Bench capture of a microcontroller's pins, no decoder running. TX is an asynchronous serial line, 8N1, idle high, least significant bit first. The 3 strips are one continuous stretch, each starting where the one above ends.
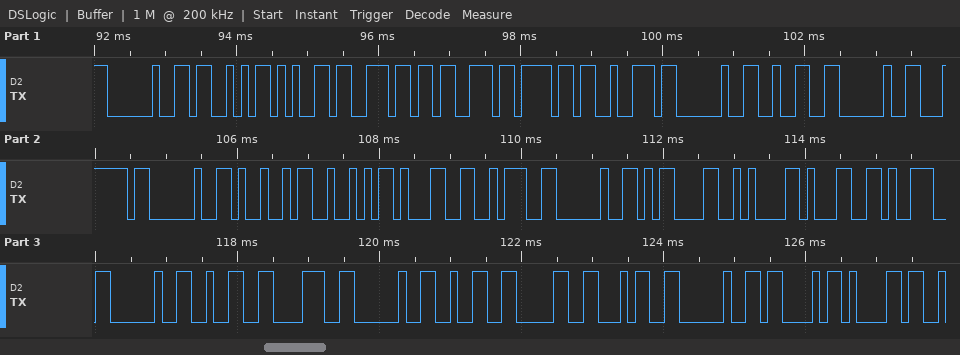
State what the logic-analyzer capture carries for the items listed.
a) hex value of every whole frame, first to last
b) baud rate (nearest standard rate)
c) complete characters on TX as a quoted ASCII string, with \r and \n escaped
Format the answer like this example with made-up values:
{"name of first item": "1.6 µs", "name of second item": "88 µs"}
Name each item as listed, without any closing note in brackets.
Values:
{"hex value of every whole frame, first to last": "20 53 65 6E 73 6F 72 20 32 20 7C 20 49 52 31 3A 20 0D 0A 31 39 20 32 38 20 32 30 34 20 43 61", "baud rate": "9600 baud", "complete characters on TX as a quoted ASCII string, with \\r and \\n escaped": "\" Sensor 2 | IR1: \\r\\n19 28 204 Ca\""}
